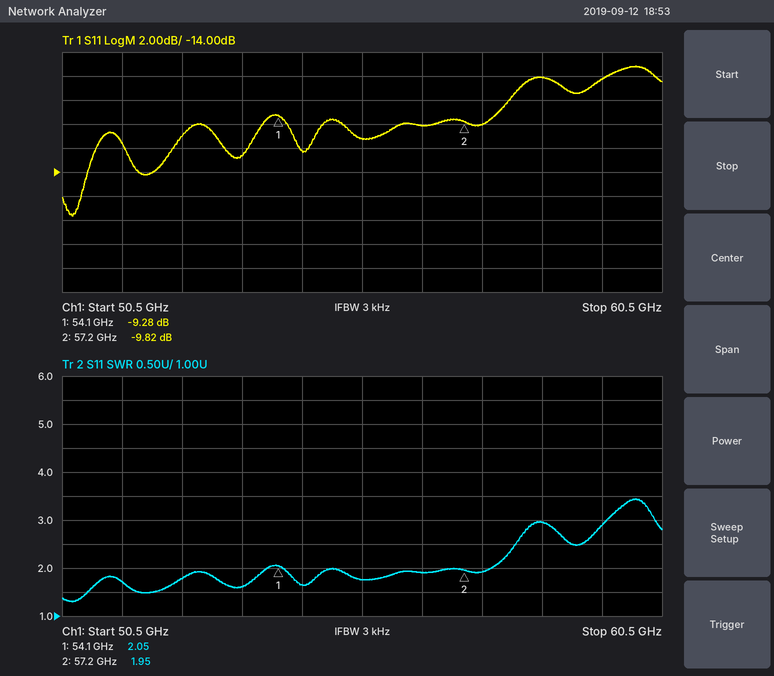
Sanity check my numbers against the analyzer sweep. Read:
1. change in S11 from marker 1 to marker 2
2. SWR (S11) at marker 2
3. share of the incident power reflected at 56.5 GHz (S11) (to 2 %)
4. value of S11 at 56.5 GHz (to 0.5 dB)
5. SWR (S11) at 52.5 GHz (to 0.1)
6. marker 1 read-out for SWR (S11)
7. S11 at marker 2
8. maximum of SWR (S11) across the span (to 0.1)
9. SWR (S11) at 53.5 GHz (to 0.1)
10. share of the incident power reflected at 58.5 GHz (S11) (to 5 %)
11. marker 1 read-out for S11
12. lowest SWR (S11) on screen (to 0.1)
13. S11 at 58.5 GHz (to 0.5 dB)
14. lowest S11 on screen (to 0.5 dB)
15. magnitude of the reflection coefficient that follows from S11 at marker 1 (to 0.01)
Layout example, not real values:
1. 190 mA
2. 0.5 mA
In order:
1. -0.54 dB
2. 1.95
3. 10 %
4. -10.0 dB
5. 1.8
6. 2.05
7. -9.82 dB
8. 3.4
9. 1.6
10. 25 %
11. -9.28 dB
12. 1.3
13. -6.0 dB
14. -17.5 dB
15. 0.34
